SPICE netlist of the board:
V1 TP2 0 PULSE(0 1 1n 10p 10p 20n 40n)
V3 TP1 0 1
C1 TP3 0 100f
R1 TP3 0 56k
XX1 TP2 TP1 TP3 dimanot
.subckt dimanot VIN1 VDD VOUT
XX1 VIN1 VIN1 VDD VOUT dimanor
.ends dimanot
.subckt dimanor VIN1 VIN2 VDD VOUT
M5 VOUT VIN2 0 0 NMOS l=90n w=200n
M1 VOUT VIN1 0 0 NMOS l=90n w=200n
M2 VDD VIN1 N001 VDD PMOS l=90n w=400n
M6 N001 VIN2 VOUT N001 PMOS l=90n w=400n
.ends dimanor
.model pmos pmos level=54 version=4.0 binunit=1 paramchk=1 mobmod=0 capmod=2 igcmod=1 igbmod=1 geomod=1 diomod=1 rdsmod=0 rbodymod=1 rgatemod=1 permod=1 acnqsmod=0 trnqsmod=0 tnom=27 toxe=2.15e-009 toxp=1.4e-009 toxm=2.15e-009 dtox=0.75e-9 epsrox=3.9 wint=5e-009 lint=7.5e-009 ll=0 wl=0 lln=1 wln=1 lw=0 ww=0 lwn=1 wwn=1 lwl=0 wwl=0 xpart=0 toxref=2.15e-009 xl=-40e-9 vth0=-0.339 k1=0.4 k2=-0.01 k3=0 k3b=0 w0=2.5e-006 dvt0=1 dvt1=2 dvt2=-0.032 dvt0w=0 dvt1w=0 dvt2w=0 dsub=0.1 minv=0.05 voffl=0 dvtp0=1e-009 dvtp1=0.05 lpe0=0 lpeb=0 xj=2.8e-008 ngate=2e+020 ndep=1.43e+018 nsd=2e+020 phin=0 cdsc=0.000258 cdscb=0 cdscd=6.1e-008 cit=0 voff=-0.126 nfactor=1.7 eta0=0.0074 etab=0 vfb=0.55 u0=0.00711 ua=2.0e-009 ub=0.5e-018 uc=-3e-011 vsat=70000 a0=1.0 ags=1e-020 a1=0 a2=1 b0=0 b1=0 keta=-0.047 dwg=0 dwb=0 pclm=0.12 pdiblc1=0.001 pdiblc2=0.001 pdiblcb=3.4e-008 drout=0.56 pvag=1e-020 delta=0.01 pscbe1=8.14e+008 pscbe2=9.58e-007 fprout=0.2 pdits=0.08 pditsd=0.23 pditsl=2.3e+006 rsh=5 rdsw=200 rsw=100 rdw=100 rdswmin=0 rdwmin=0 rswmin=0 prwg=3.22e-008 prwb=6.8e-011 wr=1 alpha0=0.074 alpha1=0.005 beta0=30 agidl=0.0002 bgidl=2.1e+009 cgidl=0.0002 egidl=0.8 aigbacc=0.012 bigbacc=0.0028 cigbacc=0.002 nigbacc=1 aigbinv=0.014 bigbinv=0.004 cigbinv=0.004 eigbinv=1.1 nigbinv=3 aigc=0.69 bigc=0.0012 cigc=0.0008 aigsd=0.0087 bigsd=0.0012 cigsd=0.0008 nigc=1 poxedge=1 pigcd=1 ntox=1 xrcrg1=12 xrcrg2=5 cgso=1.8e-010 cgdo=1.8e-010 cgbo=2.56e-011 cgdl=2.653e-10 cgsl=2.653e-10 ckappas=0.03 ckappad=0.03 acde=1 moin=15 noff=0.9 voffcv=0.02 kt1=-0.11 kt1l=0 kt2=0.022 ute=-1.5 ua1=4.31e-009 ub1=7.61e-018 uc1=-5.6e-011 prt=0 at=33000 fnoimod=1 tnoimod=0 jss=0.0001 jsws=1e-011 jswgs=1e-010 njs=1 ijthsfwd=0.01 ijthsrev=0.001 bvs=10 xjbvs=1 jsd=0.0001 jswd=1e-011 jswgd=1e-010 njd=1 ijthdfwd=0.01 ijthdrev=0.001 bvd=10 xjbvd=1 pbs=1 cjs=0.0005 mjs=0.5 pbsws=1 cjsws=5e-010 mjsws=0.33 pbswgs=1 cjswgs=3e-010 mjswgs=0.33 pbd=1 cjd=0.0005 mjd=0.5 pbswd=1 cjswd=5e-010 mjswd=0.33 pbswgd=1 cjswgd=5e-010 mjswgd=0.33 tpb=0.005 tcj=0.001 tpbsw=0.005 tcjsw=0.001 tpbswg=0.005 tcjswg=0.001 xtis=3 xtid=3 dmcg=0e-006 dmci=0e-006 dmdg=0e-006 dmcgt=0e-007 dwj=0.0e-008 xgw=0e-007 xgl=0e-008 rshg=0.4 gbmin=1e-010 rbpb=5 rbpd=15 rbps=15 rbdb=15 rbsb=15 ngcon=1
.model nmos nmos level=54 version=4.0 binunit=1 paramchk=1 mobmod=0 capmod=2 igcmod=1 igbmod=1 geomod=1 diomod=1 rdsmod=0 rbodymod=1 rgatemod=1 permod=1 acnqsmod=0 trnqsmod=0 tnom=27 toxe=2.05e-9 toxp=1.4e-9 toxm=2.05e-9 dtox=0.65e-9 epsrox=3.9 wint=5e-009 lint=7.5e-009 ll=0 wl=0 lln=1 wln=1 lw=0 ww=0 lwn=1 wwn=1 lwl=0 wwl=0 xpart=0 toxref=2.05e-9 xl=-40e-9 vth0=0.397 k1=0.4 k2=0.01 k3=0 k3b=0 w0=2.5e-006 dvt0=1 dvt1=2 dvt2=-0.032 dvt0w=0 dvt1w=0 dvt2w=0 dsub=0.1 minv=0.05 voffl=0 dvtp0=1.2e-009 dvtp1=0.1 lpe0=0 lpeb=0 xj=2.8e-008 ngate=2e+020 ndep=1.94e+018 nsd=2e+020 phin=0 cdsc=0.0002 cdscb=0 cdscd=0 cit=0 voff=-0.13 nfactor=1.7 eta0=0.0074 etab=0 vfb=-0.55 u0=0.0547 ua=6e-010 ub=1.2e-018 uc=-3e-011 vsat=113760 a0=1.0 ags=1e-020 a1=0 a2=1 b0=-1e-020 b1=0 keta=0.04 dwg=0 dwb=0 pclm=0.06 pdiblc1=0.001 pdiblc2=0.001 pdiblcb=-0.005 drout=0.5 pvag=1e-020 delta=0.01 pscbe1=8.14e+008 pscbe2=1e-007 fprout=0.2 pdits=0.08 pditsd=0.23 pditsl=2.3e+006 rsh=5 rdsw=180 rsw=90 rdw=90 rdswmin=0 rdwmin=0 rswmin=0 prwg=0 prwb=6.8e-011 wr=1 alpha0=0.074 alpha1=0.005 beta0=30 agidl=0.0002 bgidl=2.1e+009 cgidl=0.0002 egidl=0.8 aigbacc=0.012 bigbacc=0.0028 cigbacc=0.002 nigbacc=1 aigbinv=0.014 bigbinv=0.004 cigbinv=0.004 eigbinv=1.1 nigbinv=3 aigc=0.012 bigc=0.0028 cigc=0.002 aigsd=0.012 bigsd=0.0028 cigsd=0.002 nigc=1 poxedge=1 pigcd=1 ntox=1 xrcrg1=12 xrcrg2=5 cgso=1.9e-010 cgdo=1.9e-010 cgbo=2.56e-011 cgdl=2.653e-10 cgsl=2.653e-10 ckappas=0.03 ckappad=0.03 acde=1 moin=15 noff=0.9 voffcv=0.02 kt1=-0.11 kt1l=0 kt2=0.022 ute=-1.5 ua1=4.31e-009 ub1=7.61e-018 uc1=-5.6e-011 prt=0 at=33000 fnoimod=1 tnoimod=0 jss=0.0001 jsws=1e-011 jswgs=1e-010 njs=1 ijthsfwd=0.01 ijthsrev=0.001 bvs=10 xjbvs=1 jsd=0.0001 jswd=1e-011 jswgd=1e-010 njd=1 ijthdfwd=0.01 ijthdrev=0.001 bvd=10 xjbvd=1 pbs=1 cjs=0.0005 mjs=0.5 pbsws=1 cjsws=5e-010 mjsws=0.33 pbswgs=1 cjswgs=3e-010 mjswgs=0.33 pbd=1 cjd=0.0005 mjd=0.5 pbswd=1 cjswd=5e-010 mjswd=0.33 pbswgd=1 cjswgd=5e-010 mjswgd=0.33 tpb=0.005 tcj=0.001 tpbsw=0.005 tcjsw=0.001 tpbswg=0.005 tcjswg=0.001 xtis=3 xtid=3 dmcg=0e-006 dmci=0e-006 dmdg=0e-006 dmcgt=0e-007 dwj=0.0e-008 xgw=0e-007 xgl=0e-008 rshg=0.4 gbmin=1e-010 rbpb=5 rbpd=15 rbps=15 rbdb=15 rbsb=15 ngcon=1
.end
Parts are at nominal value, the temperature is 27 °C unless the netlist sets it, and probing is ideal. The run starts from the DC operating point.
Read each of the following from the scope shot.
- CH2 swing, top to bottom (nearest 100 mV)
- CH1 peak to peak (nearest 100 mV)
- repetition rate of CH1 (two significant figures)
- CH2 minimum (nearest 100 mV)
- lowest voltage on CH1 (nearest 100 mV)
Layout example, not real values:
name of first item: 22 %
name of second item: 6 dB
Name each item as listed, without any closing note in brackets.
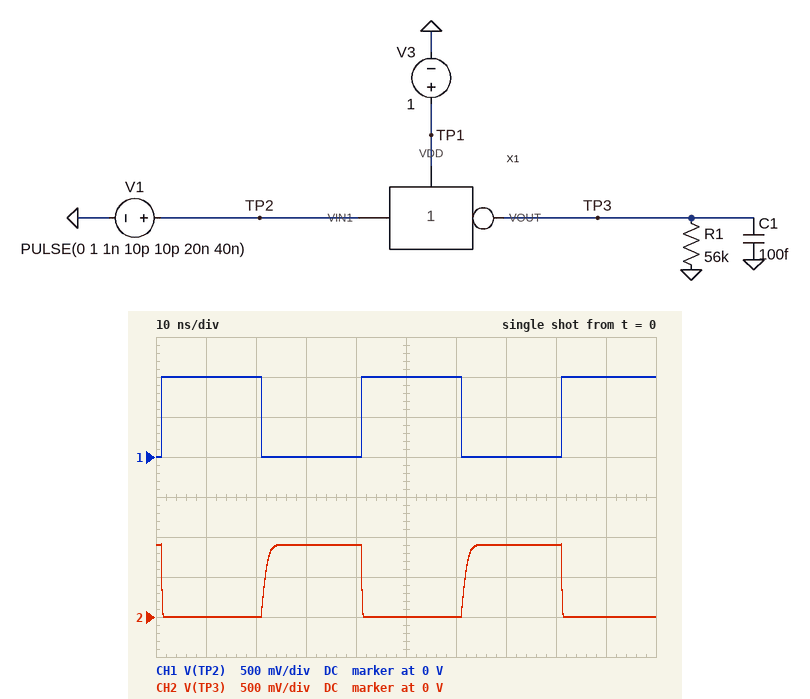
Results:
CH2 swing, top to bottom: 900 mV
CH1 peak to peak: 1.0 V
repetition rate of CH1: 25 MHz
CH2 minimum: 0 V
lowest voltage on CH1: 0 V
